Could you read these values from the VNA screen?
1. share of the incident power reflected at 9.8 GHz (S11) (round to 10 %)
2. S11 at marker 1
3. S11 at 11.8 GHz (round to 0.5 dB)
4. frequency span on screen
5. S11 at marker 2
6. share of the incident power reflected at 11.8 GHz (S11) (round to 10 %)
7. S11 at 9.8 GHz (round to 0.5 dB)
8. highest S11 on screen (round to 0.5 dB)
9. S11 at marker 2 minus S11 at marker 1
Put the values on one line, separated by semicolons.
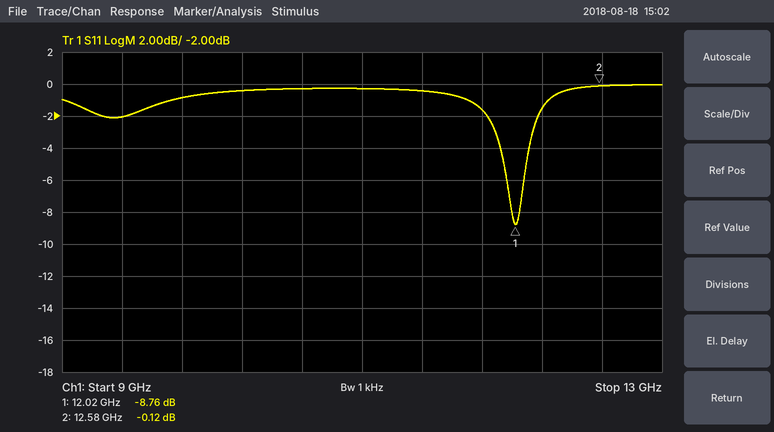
80 %; -8.76 dB; -1.5 dB; 4 GHz; -0.12 dB; 70 %; -1.0 dB; 0.0 dB; 8.64 dB
